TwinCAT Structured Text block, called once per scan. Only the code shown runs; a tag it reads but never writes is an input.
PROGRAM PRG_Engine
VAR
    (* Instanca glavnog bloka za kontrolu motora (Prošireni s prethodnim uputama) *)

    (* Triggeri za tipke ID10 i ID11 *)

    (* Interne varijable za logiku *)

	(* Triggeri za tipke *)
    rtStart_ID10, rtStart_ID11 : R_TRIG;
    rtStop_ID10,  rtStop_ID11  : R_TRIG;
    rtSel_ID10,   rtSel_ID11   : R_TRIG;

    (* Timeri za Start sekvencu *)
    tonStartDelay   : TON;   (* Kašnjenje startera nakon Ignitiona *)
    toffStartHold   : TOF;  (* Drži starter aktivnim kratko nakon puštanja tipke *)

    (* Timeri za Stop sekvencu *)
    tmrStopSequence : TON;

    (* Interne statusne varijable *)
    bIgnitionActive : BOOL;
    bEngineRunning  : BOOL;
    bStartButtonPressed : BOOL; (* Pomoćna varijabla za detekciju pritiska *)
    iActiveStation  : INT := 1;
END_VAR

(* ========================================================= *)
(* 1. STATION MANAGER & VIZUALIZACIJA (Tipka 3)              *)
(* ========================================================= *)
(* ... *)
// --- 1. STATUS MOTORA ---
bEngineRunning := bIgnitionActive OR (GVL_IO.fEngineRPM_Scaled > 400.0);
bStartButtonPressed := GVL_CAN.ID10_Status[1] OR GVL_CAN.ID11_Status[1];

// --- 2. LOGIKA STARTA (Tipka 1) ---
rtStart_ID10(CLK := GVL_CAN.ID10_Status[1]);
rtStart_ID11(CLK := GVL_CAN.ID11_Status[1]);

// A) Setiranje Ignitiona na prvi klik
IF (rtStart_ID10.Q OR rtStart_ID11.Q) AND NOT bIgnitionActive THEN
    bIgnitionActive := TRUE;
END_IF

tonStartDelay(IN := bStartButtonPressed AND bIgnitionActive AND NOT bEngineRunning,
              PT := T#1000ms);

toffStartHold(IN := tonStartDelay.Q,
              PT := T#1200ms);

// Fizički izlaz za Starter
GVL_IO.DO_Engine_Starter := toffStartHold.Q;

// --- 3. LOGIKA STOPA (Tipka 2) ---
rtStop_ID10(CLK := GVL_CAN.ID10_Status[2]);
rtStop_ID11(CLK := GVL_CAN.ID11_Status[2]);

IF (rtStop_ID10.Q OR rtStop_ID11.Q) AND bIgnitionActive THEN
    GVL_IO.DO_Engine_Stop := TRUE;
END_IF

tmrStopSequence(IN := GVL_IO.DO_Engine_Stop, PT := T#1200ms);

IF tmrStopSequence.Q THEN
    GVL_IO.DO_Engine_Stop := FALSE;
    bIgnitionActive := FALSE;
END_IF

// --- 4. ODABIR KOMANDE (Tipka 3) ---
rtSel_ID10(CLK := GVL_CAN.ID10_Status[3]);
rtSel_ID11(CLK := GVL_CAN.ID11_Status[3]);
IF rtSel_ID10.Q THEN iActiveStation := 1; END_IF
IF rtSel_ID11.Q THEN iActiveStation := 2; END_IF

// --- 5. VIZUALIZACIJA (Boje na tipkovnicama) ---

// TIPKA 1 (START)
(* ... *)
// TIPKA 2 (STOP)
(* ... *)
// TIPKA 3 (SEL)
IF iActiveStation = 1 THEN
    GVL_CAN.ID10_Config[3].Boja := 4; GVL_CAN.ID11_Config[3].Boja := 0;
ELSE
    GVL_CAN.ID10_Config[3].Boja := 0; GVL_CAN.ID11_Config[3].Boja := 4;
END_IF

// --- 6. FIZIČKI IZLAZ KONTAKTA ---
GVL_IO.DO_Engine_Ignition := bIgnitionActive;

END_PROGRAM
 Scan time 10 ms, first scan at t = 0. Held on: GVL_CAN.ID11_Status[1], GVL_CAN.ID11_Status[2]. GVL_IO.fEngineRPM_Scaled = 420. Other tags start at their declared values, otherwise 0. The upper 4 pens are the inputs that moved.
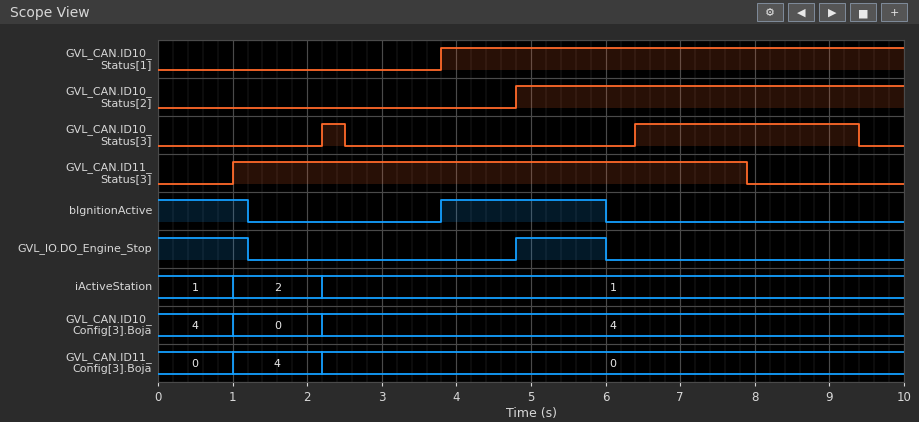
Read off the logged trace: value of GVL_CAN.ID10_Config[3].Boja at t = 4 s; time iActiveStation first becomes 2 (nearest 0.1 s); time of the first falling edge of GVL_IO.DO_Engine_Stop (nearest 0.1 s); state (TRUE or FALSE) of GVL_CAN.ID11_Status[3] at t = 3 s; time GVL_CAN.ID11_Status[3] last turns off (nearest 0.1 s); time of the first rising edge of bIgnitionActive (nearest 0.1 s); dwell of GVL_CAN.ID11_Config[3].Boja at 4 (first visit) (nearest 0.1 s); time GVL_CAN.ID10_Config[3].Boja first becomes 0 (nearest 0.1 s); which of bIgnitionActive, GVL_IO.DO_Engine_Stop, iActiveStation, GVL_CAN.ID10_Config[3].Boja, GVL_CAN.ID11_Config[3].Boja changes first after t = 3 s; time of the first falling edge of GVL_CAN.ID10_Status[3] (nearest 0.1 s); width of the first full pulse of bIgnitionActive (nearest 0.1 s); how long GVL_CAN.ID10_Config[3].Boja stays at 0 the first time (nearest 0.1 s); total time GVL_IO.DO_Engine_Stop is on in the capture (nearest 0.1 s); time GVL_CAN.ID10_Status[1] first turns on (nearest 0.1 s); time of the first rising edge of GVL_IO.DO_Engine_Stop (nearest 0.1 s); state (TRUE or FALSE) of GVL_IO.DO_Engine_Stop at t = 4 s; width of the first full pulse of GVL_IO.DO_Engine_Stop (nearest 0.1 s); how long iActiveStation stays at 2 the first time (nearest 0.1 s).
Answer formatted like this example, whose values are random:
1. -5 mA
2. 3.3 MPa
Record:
1. 4
2. 1.0 s
3. 1.2 s
4. TRUE
5. 7.9 s
6. 3.8 s
7. 1.2 s
8. 1.0 s
9. bIgnitionActive
10. 2.5 s
11. 2.2 s
12. 1.2 s
13. 2.4 s
14. 3.8 s
15. 4.8 s
16. FALSE
17. 1.2 s
18. 1.2 s
